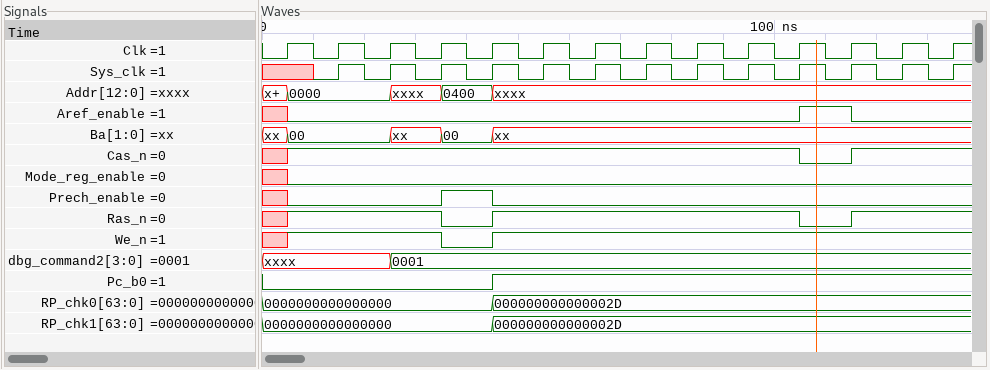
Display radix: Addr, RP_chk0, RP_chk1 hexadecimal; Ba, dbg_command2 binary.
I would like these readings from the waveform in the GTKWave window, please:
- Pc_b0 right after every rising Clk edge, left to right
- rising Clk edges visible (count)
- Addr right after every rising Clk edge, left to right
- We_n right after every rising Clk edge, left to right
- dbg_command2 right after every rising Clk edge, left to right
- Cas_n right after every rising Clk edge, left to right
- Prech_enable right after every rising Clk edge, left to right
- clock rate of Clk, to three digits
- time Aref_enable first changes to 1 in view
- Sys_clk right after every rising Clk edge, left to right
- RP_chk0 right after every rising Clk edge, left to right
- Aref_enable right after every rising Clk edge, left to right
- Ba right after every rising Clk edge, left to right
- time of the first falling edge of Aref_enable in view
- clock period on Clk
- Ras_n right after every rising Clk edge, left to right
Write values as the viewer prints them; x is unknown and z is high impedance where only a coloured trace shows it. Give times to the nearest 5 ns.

0 0 0 0 1 1 1 1 1 1 1 1 1 1
14
0000, 0000, xxxx, 0400, xxxx, xxxx, xxxx, xxxx, xxxx, xxxx, xxxx, xxxx, xxxx, xxxx
1 1 1 0 1 1 1 1 1 1 1 1 1 1
xxxx, xxxx, 0001, 0001, 0001, 0001, 0001, 0001, 0001, 0001, 0001, 0001, 0001, 0001
1 1 1 1 1 1 1 1 1 1 0 1 1 1
0 0 0 1 0 0 0 0 0 0 0 0 0 0
100 MHz
105 ns
x 1 1 1 1 1 1 1 1 1 1 1 1 1
0000000000000000, 0000000000000000, 0000000000000000, 0000000000000000, 000000000000002D, 000000000000002D, 000000000000002D, 000000000000002D, 000000000000002D, 000000000000002D, 000000000000002D, 000000000000002D, 000000000000002D, 000000000000002D
0 0 0 0 0 0 0 0 0 0 1 0 0 0
00, 00, xx, 00, xx, xx, xx, xx, xx, xx, xx, xx, xx, xx
115 ns
10 ns
1 1 1 0 1 1 1 1 1 1 0 1 1 1
